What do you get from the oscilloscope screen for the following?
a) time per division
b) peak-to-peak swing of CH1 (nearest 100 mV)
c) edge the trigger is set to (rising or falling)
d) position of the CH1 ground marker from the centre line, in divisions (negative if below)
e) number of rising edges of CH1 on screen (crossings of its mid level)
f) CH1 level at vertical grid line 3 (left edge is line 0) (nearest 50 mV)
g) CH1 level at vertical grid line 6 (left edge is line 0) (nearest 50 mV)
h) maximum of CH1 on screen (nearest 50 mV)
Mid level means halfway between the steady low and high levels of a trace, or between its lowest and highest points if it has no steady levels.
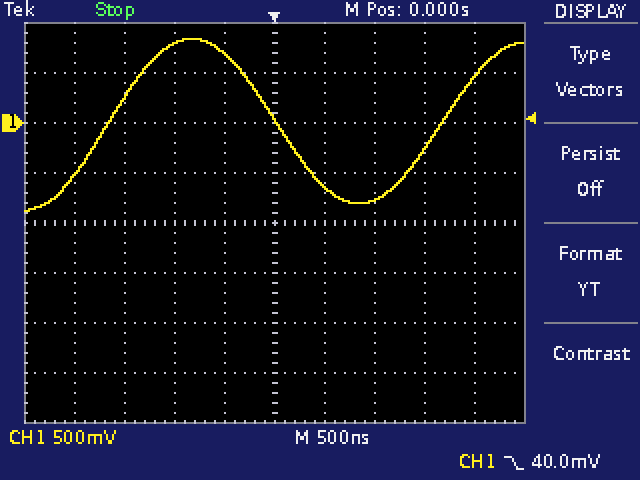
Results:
500 ns
1.70 V
falling
+2.0 div
2
800 mV
-650 mV
850 mV
